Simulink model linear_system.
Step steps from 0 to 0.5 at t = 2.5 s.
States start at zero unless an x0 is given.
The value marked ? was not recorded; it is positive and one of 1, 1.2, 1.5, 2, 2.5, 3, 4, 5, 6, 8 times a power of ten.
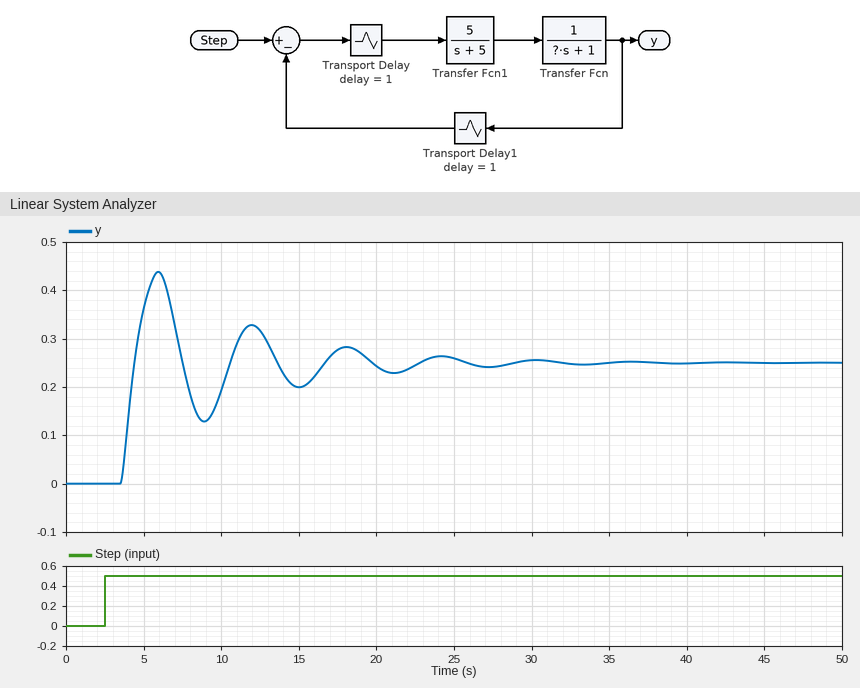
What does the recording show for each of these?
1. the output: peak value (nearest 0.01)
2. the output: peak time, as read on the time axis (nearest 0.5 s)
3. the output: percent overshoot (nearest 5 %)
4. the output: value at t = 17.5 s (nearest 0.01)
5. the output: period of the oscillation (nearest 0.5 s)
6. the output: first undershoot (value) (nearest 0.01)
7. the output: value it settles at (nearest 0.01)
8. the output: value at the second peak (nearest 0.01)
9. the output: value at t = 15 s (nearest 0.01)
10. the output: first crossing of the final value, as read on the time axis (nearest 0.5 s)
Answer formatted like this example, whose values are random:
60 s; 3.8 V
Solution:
0.44; 6.0 s; 75 %; 0.28; 6.0 s; 0.13; 0.25; 0.33; 0.20; 4.5 s
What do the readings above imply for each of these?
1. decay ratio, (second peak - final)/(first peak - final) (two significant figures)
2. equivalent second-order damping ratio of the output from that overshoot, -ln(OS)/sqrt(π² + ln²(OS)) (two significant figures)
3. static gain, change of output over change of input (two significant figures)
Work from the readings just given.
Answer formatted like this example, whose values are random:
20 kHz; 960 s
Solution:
0.42; 0.091; 0.50
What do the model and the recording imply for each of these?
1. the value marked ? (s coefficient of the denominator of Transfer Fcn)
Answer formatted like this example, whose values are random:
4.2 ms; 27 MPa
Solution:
1
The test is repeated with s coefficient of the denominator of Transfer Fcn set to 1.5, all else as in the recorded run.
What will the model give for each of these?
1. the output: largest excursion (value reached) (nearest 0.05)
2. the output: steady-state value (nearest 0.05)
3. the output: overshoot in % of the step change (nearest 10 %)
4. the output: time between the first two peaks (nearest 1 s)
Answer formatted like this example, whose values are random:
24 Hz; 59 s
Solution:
0.40; 0.25; 60 %; 7 s
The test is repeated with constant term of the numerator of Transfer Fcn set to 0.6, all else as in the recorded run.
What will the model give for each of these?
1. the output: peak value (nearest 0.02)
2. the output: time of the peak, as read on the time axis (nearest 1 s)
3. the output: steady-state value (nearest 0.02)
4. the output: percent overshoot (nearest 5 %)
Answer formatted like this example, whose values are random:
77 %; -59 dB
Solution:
0.26; 6 s; 0.18; 40 %
